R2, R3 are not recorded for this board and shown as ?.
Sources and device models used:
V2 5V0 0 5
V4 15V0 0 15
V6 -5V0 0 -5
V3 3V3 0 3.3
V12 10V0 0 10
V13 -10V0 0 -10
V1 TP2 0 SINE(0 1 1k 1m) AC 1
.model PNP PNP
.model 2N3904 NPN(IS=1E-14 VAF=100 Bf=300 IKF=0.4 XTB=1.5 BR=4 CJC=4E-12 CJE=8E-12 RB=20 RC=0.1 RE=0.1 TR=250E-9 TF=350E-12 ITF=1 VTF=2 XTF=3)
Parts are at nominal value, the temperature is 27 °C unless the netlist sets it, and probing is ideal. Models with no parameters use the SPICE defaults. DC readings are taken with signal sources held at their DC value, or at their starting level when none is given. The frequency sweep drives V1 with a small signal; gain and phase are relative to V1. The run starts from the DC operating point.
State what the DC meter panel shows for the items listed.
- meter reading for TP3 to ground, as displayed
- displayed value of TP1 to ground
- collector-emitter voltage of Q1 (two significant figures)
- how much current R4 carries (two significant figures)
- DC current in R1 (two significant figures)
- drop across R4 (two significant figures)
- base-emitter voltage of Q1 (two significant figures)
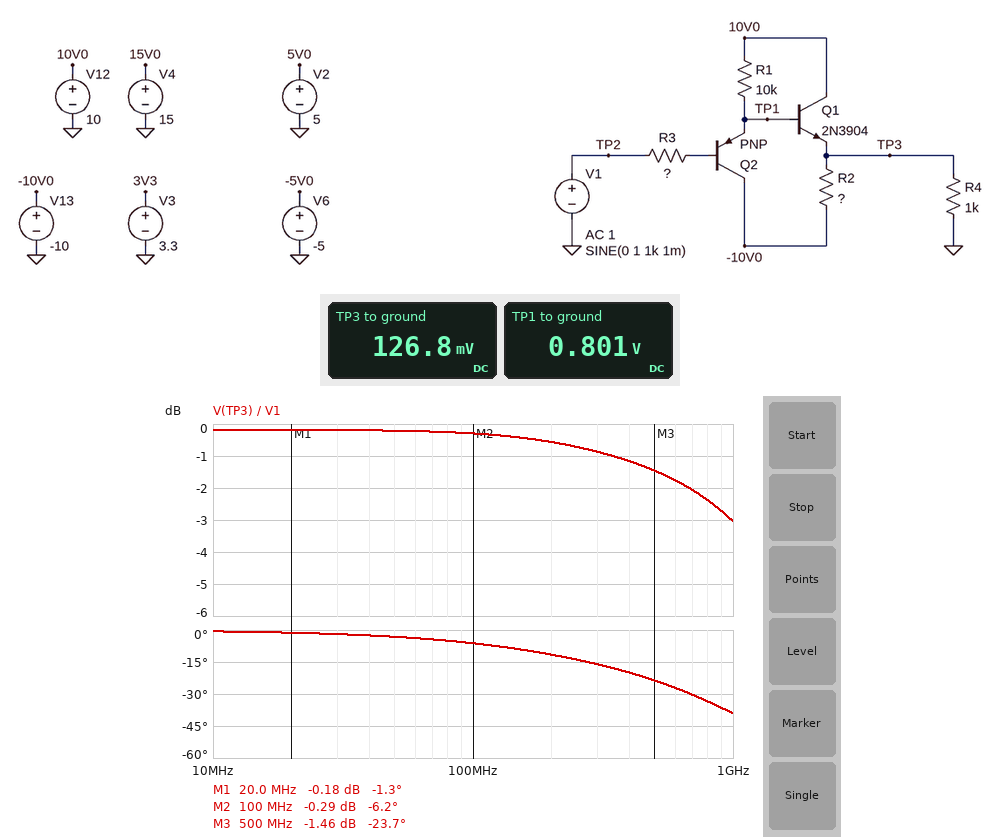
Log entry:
126.8 mV
0.801 V
9.9 V
130 µA
920 µA
130 mV
670 mV
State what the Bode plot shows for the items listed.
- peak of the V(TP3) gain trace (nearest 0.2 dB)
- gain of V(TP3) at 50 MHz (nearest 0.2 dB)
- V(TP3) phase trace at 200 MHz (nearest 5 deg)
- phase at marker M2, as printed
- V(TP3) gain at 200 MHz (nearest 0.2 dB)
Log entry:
-0.2 dB
-0.2 dB
-10 deg
-6.2 deg
-0.6 dB
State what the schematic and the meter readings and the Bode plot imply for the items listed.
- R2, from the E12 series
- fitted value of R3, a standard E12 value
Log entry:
4.7 kΩ
3.3 kΩ
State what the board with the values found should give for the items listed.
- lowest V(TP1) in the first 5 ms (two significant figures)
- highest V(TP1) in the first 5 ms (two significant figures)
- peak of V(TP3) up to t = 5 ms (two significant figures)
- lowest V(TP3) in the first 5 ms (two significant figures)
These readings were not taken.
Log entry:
-190 mV
1.8 V
1.1 V
-850 mV
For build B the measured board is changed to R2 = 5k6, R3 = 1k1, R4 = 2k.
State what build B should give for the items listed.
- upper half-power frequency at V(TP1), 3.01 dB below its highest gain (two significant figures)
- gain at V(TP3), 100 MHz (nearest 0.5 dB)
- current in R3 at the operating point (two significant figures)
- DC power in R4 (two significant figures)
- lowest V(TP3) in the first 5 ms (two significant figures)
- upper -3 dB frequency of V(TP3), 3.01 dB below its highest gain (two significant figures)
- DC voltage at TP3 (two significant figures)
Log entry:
1.8 GHz
0 dB
9.1 µA
6.3 µW
-870 mV
1.5 GHz
110 mV
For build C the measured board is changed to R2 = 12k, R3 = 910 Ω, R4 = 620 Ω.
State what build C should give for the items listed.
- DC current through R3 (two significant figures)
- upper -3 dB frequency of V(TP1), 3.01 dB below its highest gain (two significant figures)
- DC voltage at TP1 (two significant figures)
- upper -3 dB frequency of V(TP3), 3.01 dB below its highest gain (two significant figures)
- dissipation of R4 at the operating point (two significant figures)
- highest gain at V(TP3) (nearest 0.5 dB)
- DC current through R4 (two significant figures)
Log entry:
9.1 µA
1.8 GHz
780 mV
1.6 GHz
26 µW
-0.5 dB
200 µA
